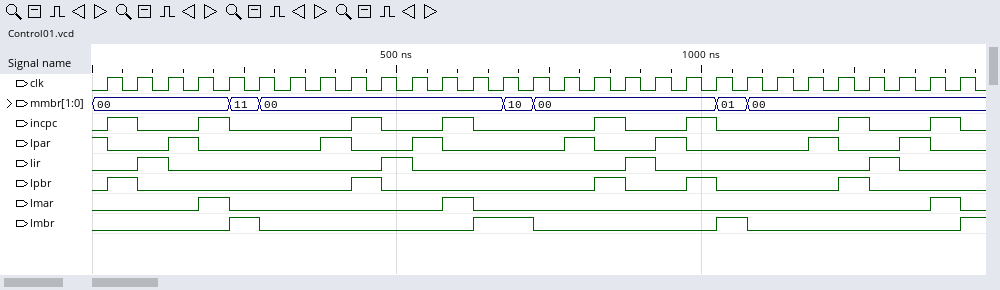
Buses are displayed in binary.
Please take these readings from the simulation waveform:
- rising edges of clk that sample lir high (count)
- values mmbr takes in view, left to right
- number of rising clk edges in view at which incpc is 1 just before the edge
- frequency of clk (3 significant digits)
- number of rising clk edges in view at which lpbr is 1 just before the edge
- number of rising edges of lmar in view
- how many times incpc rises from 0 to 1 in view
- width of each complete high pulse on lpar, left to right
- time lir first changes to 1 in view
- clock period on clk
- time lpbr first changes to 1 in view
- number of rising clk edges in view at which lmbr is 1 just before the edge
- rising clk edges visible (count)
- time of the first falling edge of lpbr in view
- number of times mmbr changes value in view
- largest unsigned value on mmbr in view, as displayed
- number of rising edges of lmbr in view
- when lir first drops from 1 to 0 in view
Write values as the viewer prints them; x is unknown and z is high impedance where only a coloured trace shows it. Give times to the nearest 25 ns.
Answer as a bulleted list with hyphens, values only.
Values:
- 4
- 00, 11, 00, 10, 00, 01, 00
- 8
- 20.0 MHz
- 5
- 3
- 8
- 50 ns, 50 ns, 50 ns, 50 ns, 50 ns, 50 ns, 50 ns
- 75 ns
- 50 ns
- 25 ns
- 4
- 29
- 75 ns
- 6
- 11
- 4
- 125 ns
